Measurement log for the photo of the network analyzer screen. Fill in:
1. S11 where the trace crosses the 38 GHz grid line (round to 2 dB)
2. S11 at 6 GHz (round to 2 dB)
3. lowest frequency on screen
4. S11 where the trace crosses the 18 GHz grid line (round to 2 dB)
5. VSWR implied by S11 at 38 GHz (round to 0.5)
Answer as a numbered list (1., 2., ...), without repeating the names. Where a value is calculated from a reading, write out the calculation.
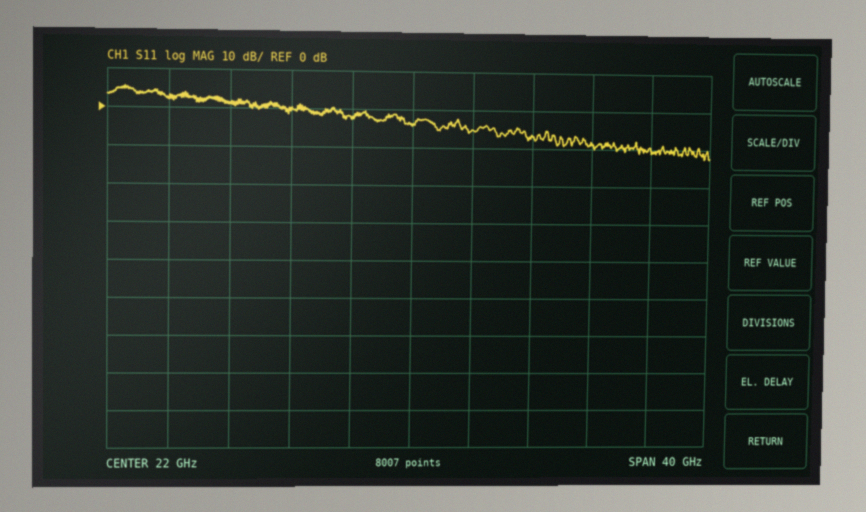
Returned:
1. -10 dB
2. 2 dB
3. 2 GHz
4. -2 dB
5. |Γ| = 10^(-10/20) = 0.3162; VSWR = (1 + 0.3162)/(1 − 0.3162) ≈ 1.92, so 2.0 to the nearest 0.5
